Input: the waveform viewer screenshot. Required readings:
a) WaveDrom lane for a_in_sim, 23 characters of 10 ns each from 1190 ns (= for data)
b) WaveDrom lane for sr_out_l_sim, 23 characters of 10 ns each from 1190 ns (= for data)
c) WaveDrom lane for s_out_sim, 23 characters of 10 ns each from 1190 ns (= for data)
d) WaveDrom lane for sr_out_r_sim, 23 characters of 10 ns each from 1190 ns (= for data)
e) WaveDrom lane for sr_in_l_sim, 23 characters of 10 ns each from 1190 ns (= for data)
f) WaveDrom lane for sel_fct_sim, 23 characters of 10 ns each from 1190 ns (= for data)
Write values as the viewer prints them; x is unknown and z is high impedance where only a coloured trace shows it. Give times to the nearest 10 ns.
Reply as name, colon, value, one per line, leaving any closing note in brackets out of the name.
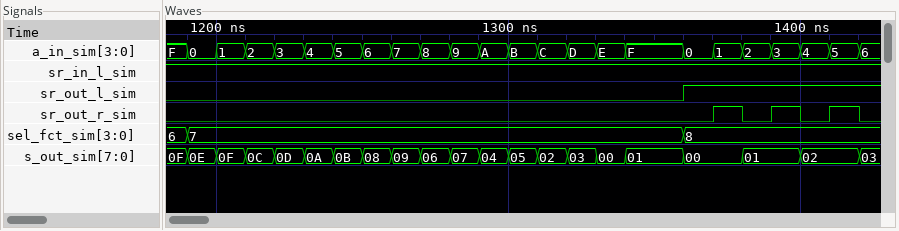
WaveDrom lane for a_in_sim, 23 characters of 10 ns each from 1190 ns: {name: 'a_in_sim', wave: '================.======', data: '0 1 2 3 4 5 6 7 8 9 A B C D E F 0 1 2 3 4 5'}
WaveDrom lane for sr_out_l_sim, 23 characters of 10 ns each from 1190 ns: {name: 'sr_out_l_sim', wave: '0................1.....'}
WaveDrom lane for s_out_sim, 23 characters of 10 ns each from 1190 ns: {name: 's_out_sim', wave: '================.=.=.=.', data: '0E 0F 0C 0D 0A 0B 08 09 06 07 04 05 02 03 00 01 00 01 02'}
WaveDrom lane for sr_out_r_sim, 23 characters of 10 ns each from 1190 ns: {name: 'sr_out_r_sim', wave: '0.................10101'}
WaveDrom lane for sr_in_l_sim, 23 characters of 10 ns each from 1190 ns: {name: 'sr_in_l_sim', wave: '1......................'}
WaveDrom lane for sel_fct_sim, 23 characters of 10 ns each from 1190 ns: {name: 'sel_fct_sim', wave: '=................=.....', data: '7 8'}
